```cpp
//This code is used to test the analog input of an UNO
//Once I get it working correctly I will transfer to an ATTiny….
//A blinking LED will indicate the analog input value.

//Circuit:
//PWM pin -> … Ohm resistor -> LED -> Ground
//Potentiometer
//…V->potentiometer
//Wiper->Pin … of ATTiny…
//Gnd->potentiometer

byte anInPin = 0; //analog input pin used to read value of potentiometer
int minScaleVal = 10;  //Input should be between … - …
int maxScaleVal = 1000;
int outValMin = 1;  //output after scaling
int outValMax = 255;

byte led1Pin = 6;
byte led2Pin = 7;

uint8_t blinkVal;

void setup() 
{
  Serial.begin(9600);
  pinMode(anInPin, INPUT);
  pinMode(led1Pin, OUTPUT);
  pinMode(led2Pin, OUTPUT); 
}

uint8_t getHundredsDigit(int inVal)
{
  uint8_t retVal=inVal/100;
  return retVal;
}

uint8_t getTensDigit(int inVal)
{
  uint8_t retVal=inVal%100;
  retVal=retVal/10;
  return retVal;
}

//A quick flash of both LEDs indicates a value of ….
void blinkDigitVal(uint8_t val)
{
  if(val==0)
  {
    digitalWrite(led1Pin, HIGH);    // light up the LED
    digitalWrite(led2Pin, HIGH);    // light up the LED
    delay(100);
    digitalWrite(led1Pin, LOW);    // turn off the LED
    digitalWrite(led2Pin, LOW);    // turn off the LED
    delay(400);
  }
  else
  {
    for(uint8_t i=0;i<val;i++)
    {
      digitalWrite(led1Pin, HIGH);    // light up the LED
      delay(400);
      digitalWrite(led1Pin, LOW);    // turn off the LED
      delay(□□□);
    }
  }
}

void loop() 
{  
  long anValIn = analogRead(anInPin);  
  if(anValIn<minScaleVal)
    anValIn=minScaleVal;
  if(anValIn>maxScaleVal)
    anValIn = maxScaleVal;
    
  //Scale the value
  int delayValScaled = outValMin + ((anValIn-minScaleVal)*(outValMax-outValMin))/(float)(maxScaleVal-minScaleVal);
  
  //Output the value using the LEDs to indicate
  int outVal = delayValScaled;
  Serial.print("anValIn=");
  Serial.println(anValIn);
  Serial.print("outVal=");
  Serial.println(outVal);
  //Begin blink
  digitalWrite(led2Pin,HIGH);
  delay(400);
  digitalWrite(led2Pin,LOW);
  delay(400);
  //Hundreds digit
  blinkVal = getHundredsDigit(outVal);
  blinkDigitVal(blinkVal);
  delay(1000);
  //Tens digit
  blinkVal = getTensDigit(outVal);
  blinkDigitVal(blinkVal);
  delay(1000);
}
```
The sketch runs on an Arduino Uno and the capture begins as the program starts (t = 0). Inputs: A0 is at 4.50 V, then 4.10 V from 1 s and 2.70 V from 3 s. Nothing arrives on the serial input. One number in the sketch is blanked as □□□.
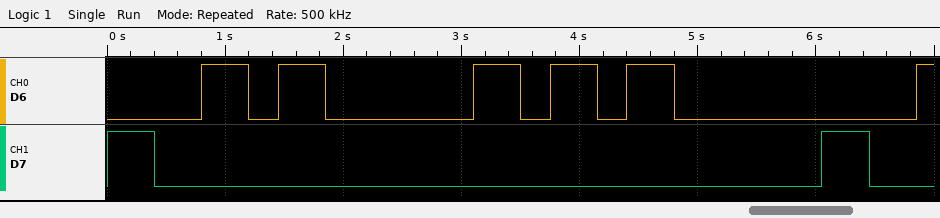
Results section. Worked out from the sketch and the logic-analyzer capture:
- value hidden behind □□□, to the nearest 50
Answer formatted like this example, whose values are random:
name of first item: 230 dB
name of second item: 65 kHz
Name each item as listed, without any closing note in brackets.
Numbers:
value hidden behind □□□, to the nearest 50: 250
